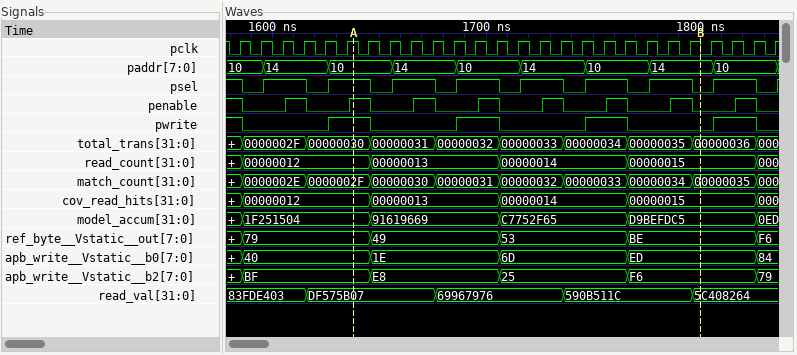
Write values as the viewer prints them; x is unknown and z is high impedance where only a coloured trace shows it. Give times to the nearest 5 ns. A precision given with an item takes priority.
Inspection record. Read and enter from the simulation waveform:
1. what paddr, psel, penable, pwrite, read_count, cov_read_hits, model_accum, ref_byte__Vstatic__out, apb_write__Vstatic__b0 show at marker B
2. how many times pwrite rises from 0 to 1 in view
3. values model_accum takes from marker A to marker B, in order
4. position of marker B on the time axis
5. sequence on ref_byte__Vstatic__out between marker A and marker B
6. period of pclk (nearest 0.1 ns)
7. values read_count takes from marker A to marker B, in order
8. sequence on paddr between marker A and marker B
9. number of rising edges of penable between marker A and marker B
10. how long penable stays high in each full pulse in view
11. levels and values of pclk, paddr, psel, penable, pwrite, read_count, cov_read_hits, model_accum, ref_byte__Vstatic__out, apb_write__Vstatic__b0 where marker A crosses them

paddr=14, psel=0, penable=0, pwrite=0, read_count=00000015, cov_read_hits=00000015, model_accum=D9BEFDC5, ref_byte__Vstatic__out=BE, apb_write__Vstatic__b0=ED
4
1F251504, 91619669, C7752F65, D9BEFDC5
1800 ns
79, 49, 53, BE
10 ns
00000012, 00000013, 00000014, 00000015
10, 14, 10, 14, 10, 14
5
10 ns, 10 ns, 10 ns, 10 ns, 10 ns, 10 ns, 10 ns, 10 ns
pclk=1, paddr=10, psel=1, penable=1, pwrite=1, read_count=00000012, cov_read_hits=00000012, model_accum=1F251504, ref_byte__Vstatic__out=79, apb_write__Vstatic__b0=40
